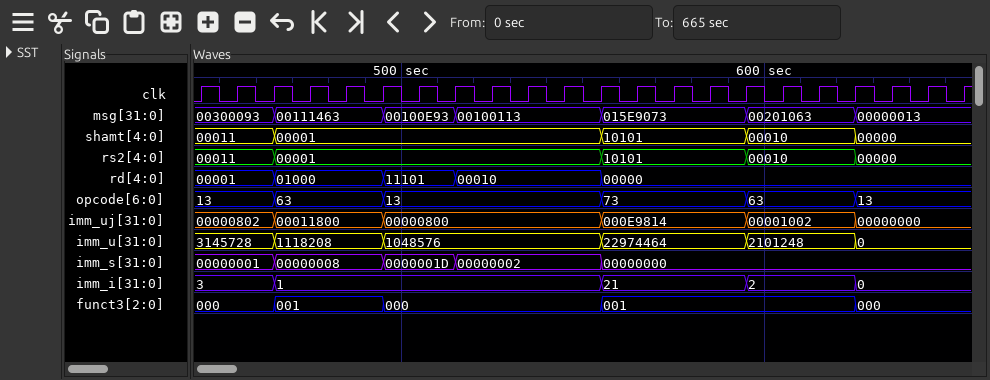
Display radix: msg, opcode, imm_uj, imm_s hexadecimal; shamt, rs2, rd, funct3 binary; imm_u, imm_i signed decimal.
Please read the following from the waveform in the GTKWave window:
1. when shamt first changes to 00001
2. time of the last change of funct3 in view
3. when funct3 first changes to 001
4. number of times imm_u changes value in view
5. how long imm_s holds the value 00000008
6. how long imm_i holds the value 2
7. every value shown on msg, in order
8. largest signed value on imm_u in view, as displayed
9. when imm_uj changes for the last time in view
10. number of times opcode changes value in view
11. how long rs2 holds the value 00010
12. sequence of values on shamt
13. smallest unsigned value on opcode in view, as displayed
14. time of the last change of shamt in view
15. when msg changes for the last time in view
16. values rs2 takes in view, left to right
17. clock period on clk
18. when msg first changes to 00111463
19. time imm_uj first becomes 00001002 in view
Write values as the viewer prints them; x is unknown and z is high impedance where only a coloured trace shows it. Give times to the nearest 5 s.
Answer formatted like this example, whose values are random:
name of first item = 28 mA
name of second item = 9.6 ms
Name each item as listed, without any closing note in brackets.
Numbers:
when shamt first changes to 00001 = 465 s
time of the last change of funct3 in view = 625 s
when funct3 first changes to 001 = 465 s
number of times imm_u changes value in view = 5
how long imm_s holds the value 00000008 = 30 s
how long imm_i holds the value 2 = 30 s
every value shown on msg, in order = 00300093, 00111463, 00100E93, 00100113, 015E9073, 00201063, 00000013
largest signed value on imm_u in view, as displayed = 22974464
when imm_uj changes for the last time in view = 625 s
number of times opcode changes value in view = 5
how long rs2 holds the value 00010 = 30 s
sequence of values on shamt = 00011, 00001, 10101, 00010, 00000
smallest unsigned value on opcode in view, as displayed = 13
time of the last change of shamt in view = 625 s
when msg changes for the last time in view = 625 s
values rs2 takes in view, left to right = 00011, 00001, 10101, 00010, 00000
clock period on clk = 10 s
when msg first changes to 00111463 = 465 s
time imm_uj first becomes 00001002 in view = 595 s
